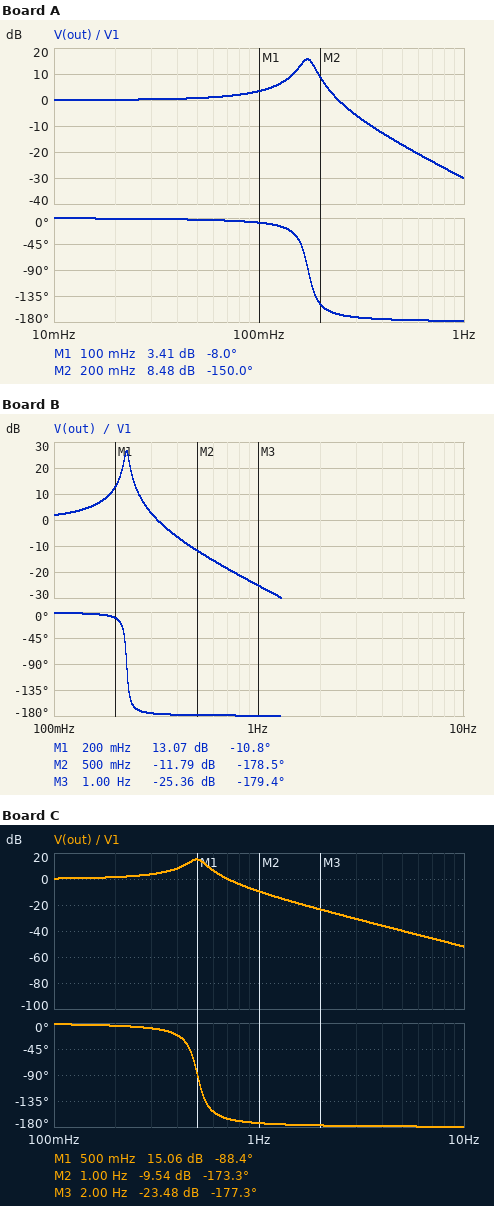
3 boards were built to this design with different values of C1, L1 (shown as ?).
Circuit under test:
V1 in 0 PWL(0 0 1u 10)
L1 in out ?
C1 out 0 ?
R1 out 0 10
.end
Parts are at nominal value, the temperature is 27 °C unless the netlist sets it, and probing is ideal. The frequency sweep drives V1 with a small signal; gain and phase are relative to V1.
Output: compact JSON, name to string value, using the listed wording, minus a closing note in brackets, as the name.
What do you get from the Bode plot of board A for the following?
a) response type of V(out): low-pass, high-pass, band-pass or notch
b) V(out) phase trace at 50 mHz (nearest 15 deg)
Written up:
{"response type of V(out): low-pass, high-pass, band-pass or notch": "low-pass", "V(out) phase trace at 50 mHz": "0 deg"}
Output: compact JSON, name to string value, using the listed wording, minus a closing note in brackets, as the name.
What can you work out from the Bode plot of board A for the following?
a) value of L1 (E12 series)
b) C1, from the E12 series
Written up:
{"value of L1": "1.5 H", "C1, from the E12 series": "560 mF"}
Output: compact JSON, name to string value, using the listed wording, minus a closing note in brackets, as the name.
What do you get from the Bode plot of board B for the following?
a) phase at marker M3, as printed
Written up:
{"phase at marker M3, as printed": "-179.4 deg"}
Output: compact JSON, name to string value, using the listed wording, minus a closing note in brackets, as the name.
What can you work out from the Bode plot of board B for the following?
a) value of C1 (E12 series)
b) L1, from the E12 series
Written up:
{"value of C1": "1.5 F", "L1, from the E12 series": "330 mH"}
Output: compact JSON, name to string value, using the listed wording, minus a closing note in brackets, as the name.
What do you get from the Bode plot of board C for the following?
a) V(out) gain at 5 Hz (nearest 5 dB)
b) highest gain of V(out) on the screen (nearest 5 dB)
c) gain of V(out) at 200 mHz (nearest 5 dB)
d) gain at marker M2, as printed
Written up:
{"V(out) gain at 5 Hz": "-40 dB", "highest gain of V(out) on the screen": "15 dB", "gain of V(out) at 200 mHz": "0 dB", "gain at marker M2, as printed": "-9.54 dB"}
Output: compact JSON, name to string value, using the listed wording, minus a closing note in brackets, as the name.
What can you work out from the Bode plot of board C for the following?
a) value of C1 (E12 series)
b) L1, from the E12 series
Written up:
{"value of C1": "180 mF", "L1, from the E12 series": "560 mH"}
